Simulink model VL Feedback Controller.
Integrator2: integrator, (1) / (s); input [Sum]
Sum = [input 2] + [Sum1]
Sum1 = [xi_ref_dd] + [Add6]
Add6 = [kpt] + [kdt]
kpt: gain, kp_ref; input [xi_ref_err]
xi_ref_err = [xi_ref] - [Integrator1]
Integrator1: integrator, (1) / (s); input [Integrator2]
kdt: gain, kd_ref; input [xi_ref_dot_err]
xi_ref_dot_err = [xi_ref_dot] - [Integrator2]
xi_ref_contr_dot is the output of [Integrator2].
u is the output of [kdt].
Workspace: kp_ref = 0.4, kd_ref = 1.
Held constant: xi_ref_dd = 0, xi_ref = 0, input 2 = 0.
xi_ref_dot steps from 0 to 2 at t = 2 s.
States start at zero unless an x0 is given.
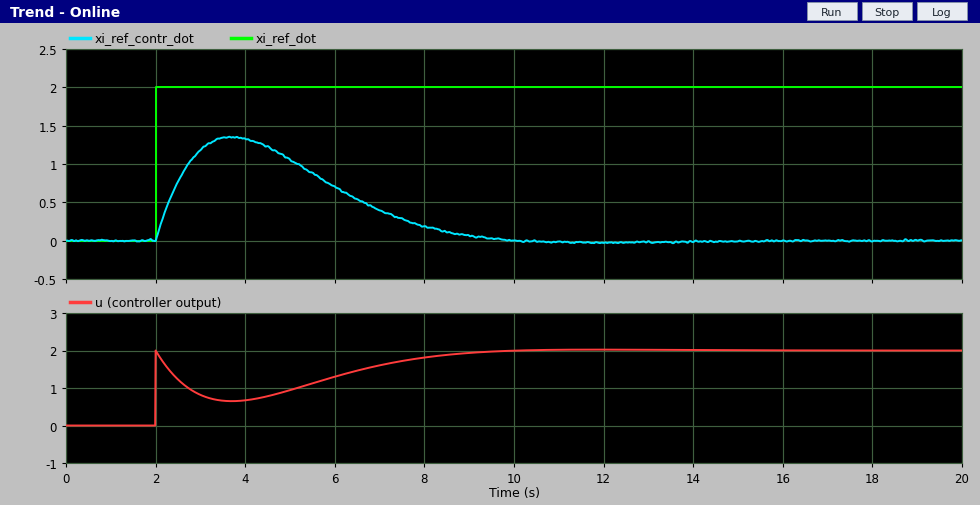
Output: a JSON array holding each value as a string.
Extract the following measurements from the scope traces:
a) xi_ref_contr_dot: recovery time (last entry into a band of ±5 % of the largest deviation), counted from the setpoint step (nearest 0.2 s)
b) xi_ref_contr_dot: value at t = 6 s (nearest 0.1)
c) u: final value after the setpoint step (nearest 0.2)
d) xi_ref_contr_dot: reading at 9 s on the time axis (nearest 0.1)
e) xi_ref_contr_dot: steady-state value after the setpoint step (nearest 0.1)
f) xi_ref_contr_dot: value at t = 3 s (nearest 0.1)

["7.0 s", "0.7", "2.0", "0.1", "0.0", "1.2"]
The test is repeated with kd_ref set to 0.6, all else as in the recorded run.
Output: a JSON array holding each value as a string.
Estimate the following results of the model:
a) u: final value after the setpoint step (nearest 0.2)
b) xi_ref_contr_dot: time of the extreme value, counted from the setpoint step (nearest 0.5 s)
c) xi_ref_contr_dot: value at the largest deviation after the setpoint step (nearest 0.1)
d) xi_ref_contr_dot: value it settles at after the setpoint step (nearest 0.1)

["1.2", "2.0 s", "1.1", "0.0"]
